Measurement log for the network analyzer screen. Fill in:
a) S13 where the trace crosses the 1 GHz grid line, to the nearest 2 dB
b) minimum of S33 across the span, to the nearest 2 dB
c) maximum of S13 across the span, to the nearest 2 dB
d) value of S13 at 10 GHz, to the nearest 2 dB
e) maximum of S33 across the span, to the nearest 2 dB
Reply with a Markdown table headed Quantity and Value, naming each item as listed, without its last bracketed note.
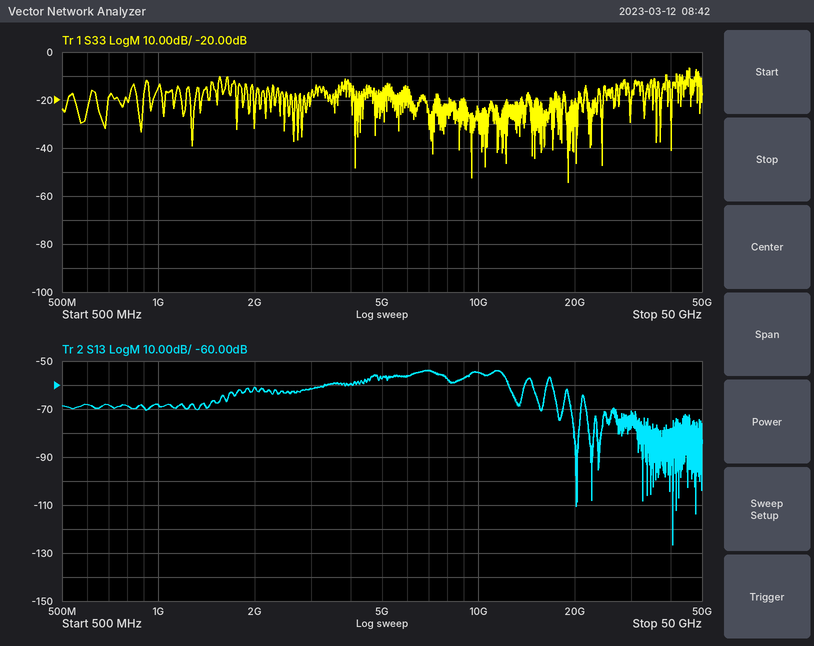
| Quantity | Value |
|---|---|
| S13 where the trace crosses the 1 GHz grid line, to the nearest 2 dB | -68 dB |
| minimum of S33 across the span, to the nearest 2 dB | -54 dB |
| maximum of S13 across the span, to the nearest 2 dB | -54 dB |
| value of S13 at 10 GHz, to the nearest 2 dB | -54 dB |
| maximum of S33 across the span, to the nearest 2 dB | -6 dB |
